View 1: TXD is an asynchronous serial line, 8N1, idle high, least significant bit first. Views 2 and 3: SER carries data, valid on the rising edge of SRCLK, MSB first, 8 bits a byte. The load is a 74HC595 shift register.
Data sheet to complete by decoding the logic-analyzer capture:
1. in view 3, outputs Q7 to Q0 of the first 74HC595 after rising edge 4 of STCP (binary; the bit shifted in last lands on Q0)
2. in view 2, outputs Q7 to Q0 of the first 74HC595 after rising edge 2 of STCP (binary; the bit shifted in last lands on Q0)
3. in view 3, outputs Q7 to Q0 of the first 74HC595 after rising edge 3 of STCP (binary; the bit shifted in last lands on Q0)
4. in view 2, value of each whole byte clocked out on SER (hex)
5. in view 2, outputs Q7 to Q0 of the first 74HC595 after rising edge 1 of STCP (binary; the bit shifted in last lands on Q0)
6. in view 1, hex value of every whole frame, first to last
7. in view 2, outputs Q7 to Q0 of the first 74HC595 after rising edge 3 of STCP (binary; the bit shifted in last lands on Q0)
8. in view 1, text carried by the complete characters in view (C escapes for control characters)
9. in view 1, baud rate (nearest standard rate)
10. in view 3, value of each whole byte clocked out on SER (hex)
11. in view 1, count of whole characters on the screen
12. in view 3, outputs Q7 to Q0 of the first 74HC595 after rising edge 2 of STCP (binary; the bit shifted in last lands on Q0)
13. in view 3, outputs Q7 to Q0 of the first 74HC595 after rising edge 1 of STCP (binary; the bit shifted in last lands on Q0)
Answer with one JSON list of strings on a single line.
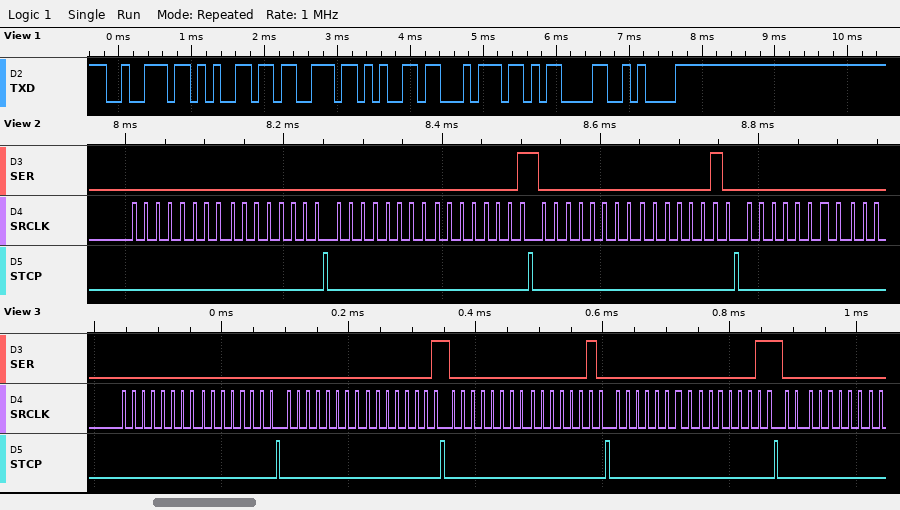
["00000011", "00000001", "00000010", "00 00 00 01 00 02 00", "00000000", "72 65 73 65 74 0D 0A", "00000010", "\"reset\\r\\n\"", "9600 baud", "00 00 00 01 00 02 00 03 00", "7", "00000001", "00000000"]
